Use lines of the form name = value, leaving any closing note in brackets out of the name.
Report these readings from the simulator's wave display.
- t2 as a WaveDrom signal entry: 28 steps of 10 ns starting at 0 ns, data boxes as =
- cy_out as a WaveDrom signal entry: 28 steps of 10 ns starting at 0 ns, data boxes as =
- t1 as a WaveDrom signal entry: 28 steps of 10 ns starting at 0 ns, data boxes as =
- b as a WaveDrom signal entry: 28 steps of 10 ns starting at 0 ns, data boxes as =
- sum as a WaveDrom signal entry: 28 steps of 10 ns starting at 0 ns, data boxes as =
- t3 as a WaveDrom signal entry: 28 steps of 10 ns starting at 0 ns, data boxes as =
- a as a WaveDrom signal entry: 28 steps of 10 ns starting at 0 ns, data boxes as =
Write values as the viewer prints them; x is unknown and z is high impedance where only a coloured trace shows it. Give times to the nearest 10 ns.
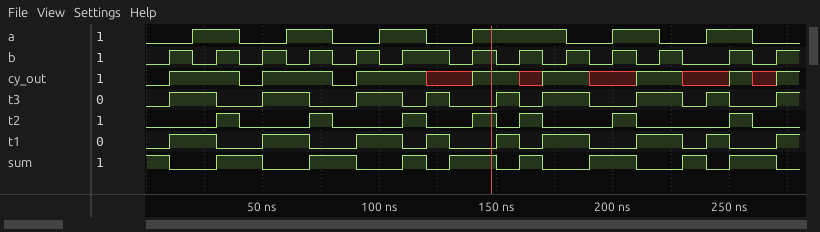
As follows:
t2 as a WaveDrom signal entry: 28 steps of 10 ns starting at 0 ns, data boxes as = = {name: 't2', wave: '0..10..10..10.1010..10...10.'}
cy_out as a WaveDrom signal entry: 28 steps of 10 ns starting at 0 ns, data boxes as = = {name: 'cy_out', wave: '01..01..01..x.1.x1.x.1.x.1x1'}
t1 as a WaveDrom signal entry: 28 steps of 10 ns starting at 0 ns, data boxes as = = {name: 't1', wave: '01.0.1.0.1.010.101.0.1.010.1'}
b as a WaveDrom signal entry: 28 steps of 10 ns starting at 0 ns, data boxes as = = {name: 'b', wave: '010101010101.01010101010.101'}
sum as a WaveDrom signal entry: 28 steps of 10 ns starting at 0 ns, data boxes as = = {name: 'sum', wave: '10.1.0.1.0.101.010.1.0.101.0'}
t3 as a WaveDrom signal entry: 28 steps of 10 ns starting at 0 ns, data boxes as = = {name: 't3', wave: '01.0.1.0.1.010.101.0.1.010.1'}
a as a WaveDrom signal entry: 28 steps of 10 ns starting at 0 ns, data boxes as = = {name: 'a', wave: '0.1.0.1.0.1.0.1...0.1.0.1.0.'}
